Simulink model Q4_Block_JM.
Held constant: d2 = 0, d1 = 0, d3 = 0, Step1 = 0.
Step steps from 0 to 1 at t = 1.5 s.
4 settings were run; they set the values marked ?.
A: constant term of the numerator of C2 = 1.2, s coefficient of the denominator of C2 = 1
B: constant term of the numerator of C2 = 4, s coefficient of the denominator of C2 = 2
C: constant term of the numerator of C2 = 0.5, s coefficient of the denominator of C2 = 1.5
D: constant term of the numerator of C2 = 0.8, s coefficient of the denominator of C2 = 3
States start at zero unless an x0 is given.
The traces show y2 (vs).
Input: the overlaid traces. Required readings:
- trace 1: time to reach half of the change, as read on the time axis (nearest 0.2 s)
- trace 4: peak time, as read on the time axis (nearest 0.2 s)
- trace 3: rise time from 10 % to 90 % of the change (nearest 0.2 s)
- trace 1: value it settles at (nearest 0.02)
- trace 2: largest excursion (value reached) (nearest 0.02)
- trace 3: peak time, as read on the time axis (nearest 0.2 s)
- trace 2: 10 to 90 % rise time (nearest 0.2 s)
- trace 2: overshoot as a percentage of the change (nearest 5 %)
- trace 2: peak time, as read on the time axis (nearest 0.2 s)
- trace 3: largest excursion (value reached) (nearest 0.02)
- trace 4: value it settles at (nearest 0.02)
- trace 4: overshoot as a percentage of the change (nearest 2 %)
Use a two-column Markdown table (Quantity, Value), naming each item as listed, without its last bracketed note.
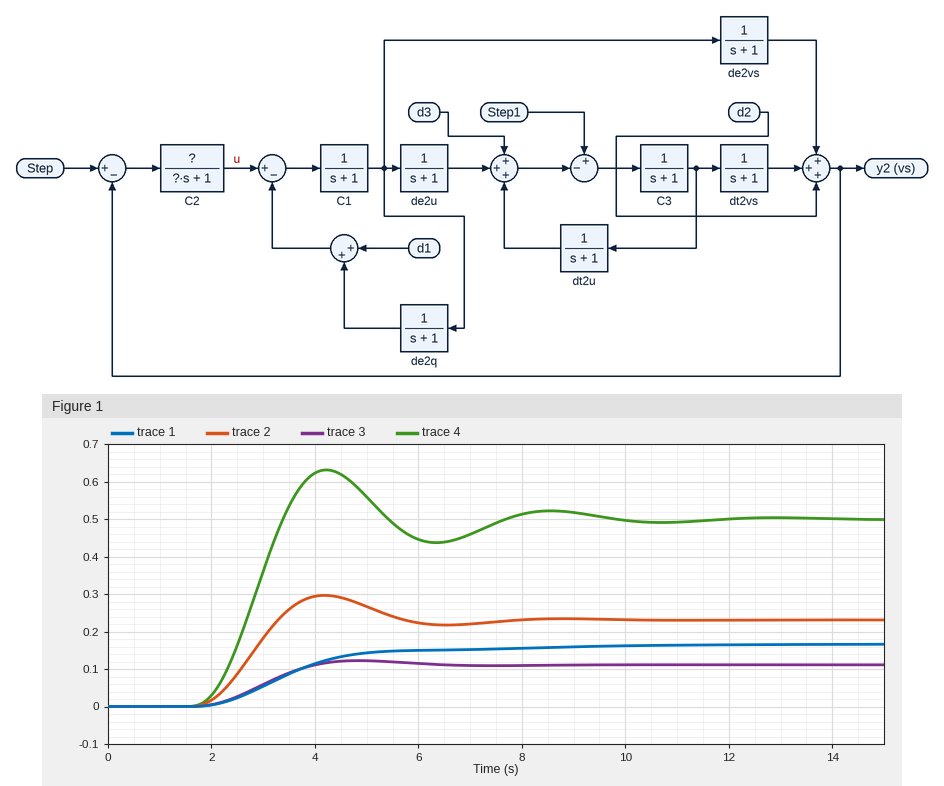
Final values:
| Quantity | Value |
|---|---|
| trace 1: time to reach half of the change, as read on the time axis | 3.4 s |
| trace 4: peak time, as read on the time axis | 4.2 s |
| trace 3: rise time from 10 % to 90 % of the change | 1.6 s |
| trace 1: value it settles at | 0.16 |
| trace 2: largest excursion (value reached) | 0.30 |
| trace 3: peak time, as read on the time axis | 4.8 s |
| trace 2: 10 to 90 % rise time | 1.0 s |
| trace 2: overshoot as a percentage of the change | 30 % |
| trace 2: peak time, as read on the time axis | 4.2 s |
| trace 3: largest excursion (value reached) | 0.12 |
| trace 4: value it settles at | 0.50 |
| trace 4: overshoot as a percentage of the change | 26 % |
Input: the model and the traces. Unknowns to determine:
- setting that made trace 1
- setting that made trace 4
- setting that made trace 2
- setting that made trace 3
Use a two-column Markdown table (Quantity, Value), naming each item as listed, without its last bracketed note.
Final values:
| Quantity | Value |
|---|---|
| setting that made trace 1 | D |
| setting that made trace 4 | B |
| setting that made trace 2 | A |
| setting that made trace 3 | C |
